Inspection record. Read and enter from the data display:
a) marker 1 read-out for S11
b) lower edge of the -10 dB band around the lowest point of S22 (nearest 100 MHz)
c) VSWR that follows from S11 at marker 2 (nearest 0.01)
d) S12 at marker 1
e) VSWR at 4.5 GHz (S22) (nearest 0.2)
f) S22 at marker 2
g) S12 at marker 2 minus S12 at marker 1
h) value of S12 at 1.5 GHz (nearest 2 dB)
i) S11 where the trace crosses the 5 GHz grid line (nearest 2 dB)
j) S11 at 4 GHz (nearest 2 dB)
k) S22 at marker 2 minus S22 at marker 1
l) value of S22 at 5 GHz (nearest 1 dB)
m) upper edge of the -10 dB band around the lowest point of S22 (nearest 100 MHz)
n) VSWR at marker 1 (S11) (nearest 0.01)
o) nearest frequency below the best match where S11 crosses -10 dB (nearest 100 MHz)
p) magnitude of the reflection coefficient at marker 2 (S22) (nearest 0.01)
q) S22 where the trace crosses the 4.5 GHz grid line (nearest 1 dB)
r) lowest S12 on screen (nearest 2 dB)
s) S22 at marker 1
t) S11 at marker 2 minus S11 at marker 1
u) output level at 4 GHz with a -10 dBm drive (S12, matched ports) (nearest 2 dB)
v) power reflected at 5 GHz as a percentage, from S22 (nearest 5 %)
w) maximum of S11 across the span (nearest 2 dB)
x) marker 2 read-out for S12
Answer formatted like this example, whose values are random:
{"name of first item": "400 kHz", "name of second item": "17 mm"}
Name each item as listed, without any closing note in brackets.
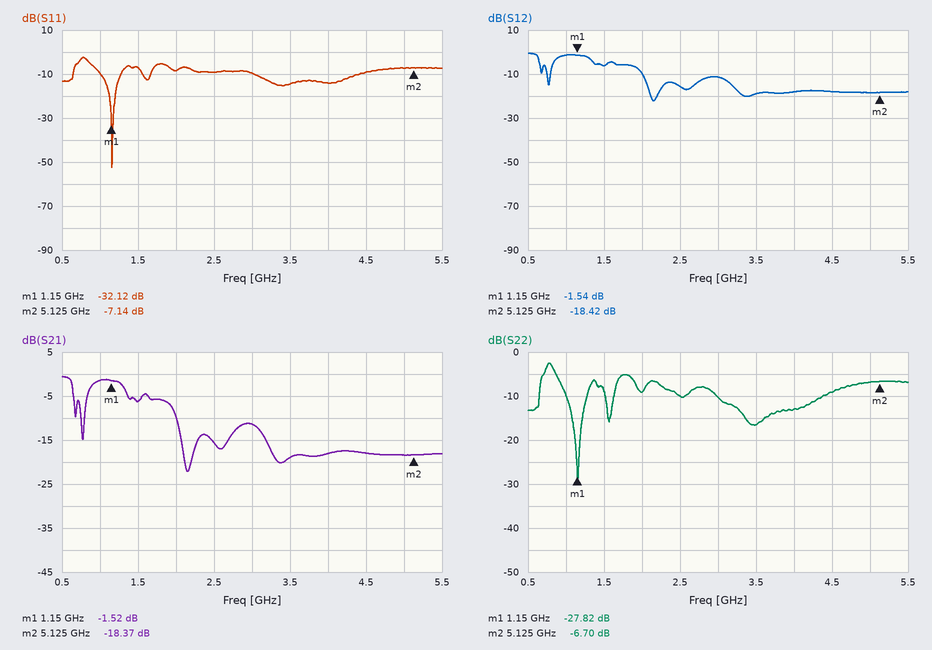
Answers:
{"marker 1 read-out for S11": "-32.12 dB", "lower edge of the -10 dB band around the lowest point of S22": "1.0 GHz", "VSWR that follows from S11 at marker 2": "2.57", "S12 at marker 1": "-1.54 dB", "VSWR at 4.5 GHz (S22)": "2.0", "S22 at marker 2": "-6.70 dB", "S12 at marker 2 minus S12 at marker 1": "-16.88 dB", "value of S12 at 1.5 GHz": "-6 dB", "S11 where the trace crosses the 5 GHz grid line": "-8 dB", "S11 at 4 GHz": "-14 dB", "S22 at marker 2 minus S22 at marker 1": "21.12 dB", "value of S22 at 5 GHz": "-7 dB", "upper edge of the -10 dB band around the lowest point of S22": "1.3 GHz", "VSWR at marker 1 (S11)": "1.05", "nearest frequency below the best match where S11 crosses -10 dB": "1.0 GHz", "magnitude of the reflection coefficient at marker 2 (S22)": "0.46", "S22 where the trace crosses the 4.5 GHz grid line": "-9 dB", "lowest S12 on screen": "-22 dB", "S22 at marker 1": "-27.82 dB", "S11 at marker 2 minus S11 at marker 1": "24.98 dB", "output level at 4 GHz with a -10 dBm drive (S12, matched ports)": "-28 dBm", "power reflected at 5 GHz as a percentage, from S22": "20 %", "maximum of S11 across the span": "-2 dB", "marker 2 read-out for S12": "-18.42 dB"}
